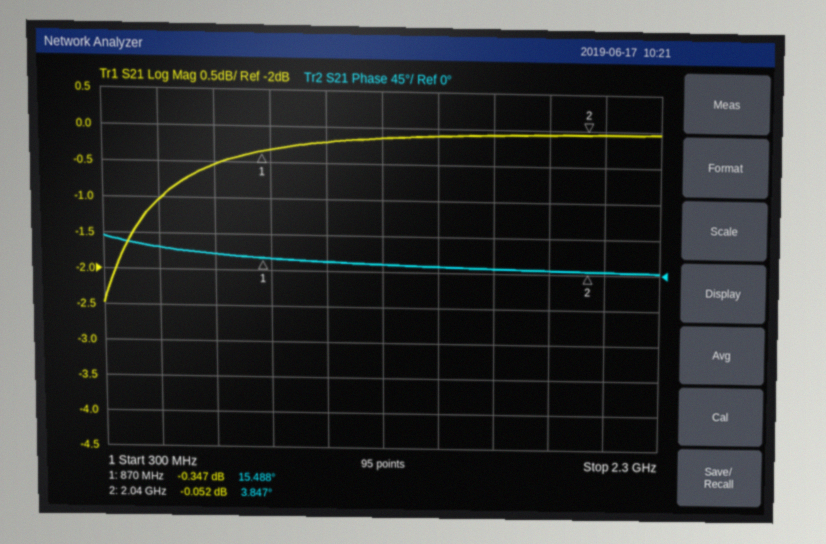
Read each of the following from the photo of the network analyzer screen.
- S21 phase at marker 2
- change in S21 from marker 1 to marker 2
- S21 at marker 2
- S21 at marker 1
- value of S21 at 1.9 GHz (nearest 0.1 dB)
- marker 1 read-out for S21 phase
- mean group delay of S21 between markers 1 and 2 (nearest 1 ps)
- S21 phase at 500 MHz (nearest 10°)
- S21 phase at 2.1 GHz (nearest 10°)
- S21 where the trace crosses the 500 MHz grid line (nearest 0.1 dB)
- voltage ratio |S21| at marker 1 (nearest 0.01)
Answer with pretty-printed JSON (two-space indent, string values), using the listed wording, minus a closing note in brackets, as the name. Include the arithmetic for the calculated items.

{
  "S21 phase at marker 2": "3.847°",
  "change in S21 from marker 1 to marker 2": "-0.052 − (-0.347) = 0.295 dB",
  "S21 at marker 2": "-0.052 dB",
  "S21 at marker 1": "-0.347 dB",
  "value of S21 at 1.9 GHz": "-0.1 dB",
  "marker 1 read-out for S21 phase": "15.488°",
  "mean group delay of S21 between markers 1 and 2": "−(3.847° − (15.488°))/(360° × 1.17 GHz) ≈ 28 ps",
  "S21 phase at 500 MHz": "30°",
  "S21 phase at 2.1 GHz": "0°",
  "S21 where the trace crosses the 500 MHz grid line": "-1.0 dB",
  "voltage ratio |S21| at marker 1": "10^(-0.347/20) ≈ 0.96"
}
